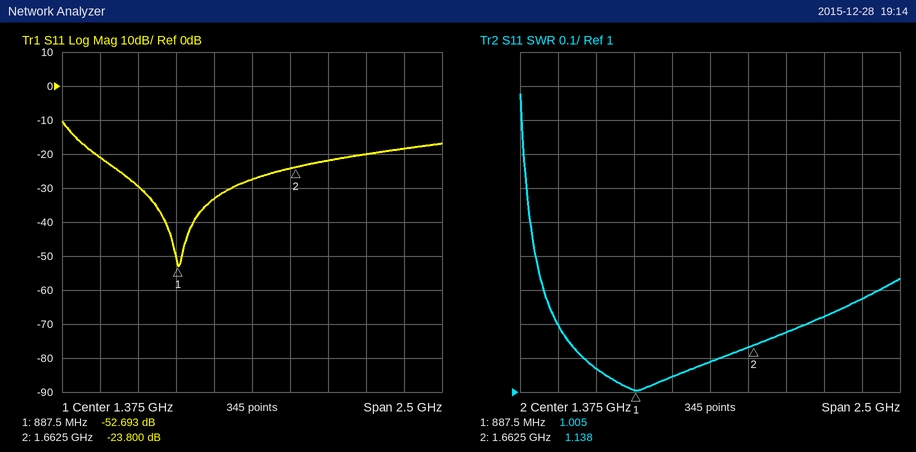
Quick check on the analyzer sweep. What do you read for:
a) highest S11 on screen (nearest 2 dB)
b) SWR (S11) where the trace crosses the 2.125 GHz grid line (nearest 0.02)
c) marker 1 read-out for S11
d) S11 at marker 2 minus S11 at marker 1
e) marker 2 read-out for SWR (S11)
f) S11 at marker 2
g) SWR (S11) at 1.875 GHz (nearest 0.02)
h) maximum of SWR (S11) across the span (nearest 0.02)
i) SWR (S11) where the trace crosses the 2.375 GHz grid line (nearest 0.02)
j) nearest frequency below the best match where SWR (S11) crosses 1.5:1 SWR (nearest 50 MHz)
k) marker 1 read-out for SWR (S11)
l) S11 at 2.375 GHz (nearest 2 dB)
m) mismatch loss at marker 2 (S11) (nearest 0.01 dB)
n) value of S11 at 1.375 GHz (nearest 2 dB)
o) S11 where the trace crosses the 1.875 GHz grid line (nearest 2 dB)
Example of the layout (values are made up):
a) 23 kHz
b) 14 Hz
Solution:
a) -10 dB
b) 1.22
c) -52.693 dB
d) 28.893 dB
e) 1.138
f) -23.800 dB
g) 1.18
h) 1.88
i) 1.28
j) 200 MHz
k) 1.005
l) -18 dB
m) 0.02 dB
n) -28 dB
o) -22 dB
